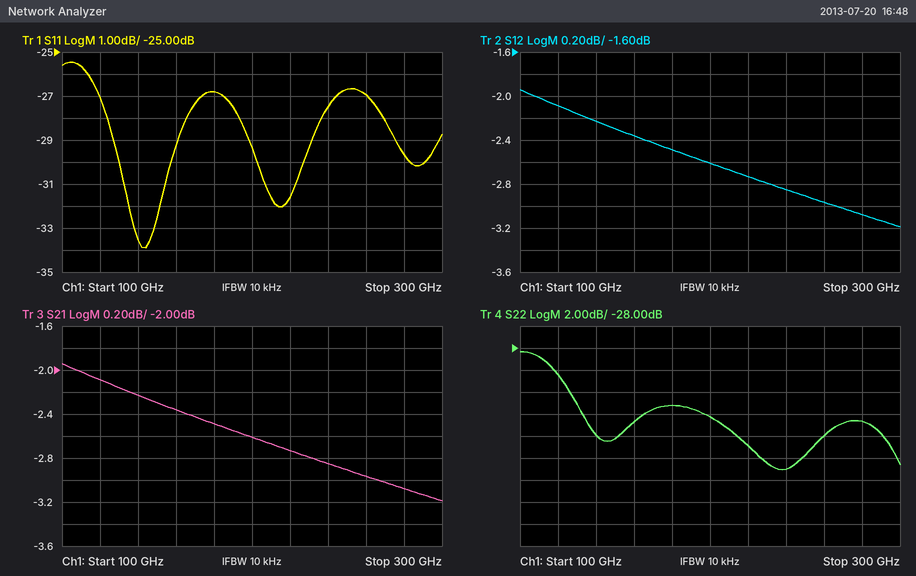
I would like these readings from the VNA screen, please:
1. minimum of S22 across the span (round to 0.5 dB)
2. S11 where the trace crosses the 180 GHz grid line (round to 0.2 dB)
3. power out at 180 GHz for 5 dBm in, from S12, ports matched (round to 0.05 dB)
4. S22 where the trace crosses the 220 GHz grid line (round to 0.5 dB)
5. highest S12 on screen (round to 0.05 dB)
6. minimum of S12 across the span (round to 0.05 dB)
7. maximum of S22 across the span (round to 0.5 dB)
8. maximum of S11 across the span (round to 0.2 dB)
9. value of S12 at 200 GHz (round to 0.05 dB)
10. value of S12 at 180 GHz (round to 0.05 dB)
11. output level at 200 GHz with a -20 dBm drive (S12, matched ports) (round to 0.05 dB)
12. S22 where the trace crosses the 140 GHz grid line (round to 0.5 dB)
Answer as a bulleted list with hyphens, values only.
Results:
- -39.0 dB
- -26.8 dB
- 2.50 dBm
- -37.0 dB
- -1.95 dB
- -3.20 dB
- -28.5 dB
- -25.4 dB
- -2.60 dB
- -2.50 dB
- -22.60 dBm
- -36.0 dB
